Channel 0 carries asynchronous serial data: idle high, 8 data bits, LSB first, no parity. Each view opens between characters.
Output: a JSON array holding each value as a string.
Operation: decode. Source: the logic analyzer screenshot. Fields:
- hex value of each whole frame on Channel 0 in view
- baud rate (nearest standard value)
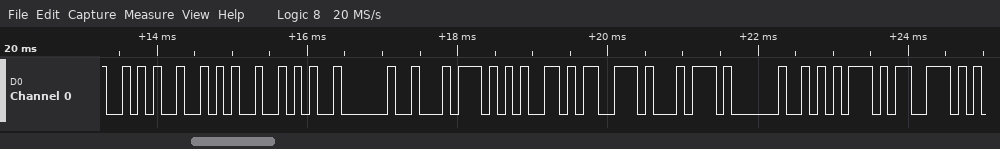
["2A, 2A, 2A, 20, 74, 65, 73, 74, 20, 75, 73", "9600 baud"]
